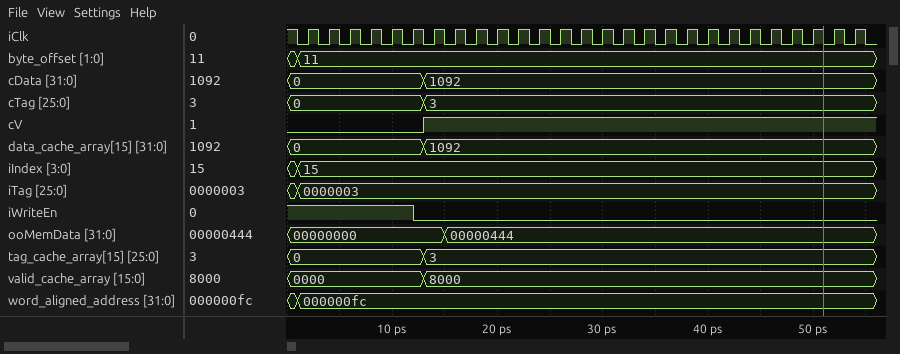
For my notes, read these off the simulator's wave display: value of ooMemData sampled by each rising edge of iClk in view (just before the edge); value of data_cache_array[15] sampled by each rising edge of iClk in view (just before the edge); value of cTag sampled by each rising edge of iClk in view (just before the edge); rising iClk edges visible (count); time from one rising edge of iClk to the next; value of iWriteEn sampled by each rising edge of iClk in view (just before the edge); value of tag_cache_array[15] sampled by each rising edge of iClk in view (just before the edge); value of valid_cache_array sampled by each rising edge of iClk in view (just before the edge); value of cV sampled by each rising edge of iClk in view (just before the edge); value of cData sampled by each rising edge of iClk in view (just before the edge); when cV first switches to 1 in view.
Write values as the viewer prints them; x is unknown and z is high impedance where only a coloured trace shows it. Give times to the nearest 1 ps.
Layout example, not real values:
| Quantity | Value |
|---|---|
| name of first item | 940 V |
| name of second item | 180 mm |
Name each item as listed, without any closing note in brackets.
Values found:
| Quantity | Value |
|---|---|
| value of ooMemData sampled by each rising edge of iClk in view | 00000000, 00000000, 00000000, 00000000, 00000000, 00000000, 00000000, 00000444, 00000444, 00000444, 00000444, 00000444, 00000444, 00000444, 00000444, 00000444, 00000444, 00000444, 00000444, 00000444, 00000444, 00000444, 00000444, 00000444, 00000444, 00000444, 00000444 |
| value of data_cache_array[15] sampled by each rising edge of iClk in view | 0, 0, 0, 0, 0, 0, 1092, 1092, 1092, 1092, 1092, 1092, 1092, 1092, 1092, 1092, 1092, 1092, 1092, 1092, 1092, 1092, 1092, 1092, 1092, 1092, 1092 |
| value of cTag sampled by each rising edge of iClk in view | 0, 0, 0, 0, 0, 0, 3, 3, 3, 3, 3, 3, 3, 3, 3, 3, 3, 3, 3, 3, 3, 3, 3, 3, 3, 3, 3 |
| rising iClk edges visible | 27 |
| time from one rising edge of iClk to the next | 2 ps |
| value of iWriteEn sampled by each rising edge of iClk in view | 1 1 1 1 1 1 0 0 0 0 0 0 0 0 0 0 0 0 0 0 0 0 0 0 0 0 0 |
| value of tag_cache_array[15] sampled by each rising edge of iClk in view | 0, 0, 0, 0, 0, 0, 3, 3, 3, 3, 3, 3, 3, 3, 3, 3, 3, 3, 3, 3, 3, 3, 3, 3, 3, 3, 3 |
| value of valid_cache_array sampled by each rising edge of iClk in view | 0000, 0000, 0000, 0000, 0000, 0000, 8000, 8000, 8000, 8000, 8000, 8000, 8000, 8000, 8000, 8000, 8000, 8000, 8000, 8000, 8000, 8000, 8000, 8000, 8000, 8000, 8000 |
| value of cV sampled by each rising edge of iClk in view | 0 0 0 0 0 0 1 1 1 1 1 1 1 1 1 1 1 1 1 1 1 1 1 1 1 1 1 |
| value of cData sampled by each rising edge of iClk in view | 0, 0, 0, 0, 0, 0, 1092, 1092, 1092, 1092, 1092, 1092, 1092, 1092, 1092, 1092, 1092, 1092, 1092, 1092, 1092, 1092, 1092, 1092, 1092, 1092, 1092 |
| when cV first switches to 1 in view | 13 ps |
